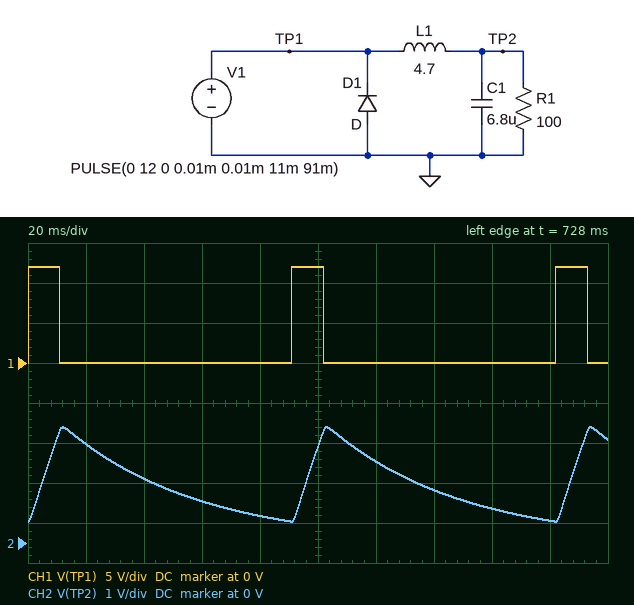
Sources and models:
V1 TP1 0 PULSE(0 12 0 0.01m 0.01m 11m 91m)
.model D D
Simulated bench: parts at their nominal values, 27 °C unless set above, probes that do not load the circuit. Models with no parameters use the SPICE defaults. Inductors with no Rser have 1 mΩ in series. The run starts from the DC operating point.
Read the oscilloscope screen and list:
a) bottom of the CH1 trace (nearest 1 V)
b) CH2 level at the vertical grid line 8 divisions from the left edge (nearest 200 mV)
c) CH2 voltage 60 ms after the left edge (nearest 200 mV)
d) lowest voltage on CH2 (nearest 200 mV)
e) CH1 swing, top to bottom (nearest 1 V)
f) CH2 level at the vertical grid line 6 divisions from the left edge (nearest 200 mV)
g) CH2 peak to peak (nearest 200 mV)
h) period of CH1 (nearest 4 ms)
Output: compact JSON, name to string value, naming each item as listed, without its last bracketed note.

{"bottom of the CH1 trace": "0 V", "CH2 level at the vertical grid line 8 divisions from the left edge": "800 mV", "CH2 voltage 60 ms after the left edge": "1.0 V", "lowest voltage on CH2": "600 mV", "CH1 swing, top to bottom": "12 V", "CH2 level at the vertical grid line 6 divisions from the left edge": "2.0 V", "CH2 peak to peak": "2.4 V", "period of CH1": "92 ms"}
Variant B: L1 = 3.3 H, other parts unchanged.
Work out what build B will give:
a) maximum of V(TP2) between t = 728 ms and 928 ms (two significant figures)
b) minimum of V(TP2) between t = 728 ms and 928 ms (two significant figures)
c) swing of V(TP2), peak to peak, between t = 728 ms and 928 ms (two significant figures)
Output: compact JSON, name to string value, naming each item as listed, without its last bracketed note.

{"maximum of V(TP2) between t = 728 ms and 928 ms": "3.6 V", "minimum of V(TP2) between t = 728 ms and 928 ms": "320 mV", "swing of V(TP2), peak to peak, between t = 728 ms and 928 ms": "3.3 V"}
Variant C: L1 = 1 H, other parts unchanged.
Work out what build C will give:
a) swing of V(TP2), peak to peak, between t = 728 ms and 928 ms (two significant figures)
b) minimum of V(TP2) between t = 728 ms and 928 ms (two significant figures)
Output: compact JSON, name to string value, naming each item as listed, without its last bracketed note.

{"swing of V(TP2), peak to peak, between t = 728 ms and 928 ms": "8.1 V", "minimum of V(TP2) between t = 728 ms and 928 ms": "1.6 mV"}
